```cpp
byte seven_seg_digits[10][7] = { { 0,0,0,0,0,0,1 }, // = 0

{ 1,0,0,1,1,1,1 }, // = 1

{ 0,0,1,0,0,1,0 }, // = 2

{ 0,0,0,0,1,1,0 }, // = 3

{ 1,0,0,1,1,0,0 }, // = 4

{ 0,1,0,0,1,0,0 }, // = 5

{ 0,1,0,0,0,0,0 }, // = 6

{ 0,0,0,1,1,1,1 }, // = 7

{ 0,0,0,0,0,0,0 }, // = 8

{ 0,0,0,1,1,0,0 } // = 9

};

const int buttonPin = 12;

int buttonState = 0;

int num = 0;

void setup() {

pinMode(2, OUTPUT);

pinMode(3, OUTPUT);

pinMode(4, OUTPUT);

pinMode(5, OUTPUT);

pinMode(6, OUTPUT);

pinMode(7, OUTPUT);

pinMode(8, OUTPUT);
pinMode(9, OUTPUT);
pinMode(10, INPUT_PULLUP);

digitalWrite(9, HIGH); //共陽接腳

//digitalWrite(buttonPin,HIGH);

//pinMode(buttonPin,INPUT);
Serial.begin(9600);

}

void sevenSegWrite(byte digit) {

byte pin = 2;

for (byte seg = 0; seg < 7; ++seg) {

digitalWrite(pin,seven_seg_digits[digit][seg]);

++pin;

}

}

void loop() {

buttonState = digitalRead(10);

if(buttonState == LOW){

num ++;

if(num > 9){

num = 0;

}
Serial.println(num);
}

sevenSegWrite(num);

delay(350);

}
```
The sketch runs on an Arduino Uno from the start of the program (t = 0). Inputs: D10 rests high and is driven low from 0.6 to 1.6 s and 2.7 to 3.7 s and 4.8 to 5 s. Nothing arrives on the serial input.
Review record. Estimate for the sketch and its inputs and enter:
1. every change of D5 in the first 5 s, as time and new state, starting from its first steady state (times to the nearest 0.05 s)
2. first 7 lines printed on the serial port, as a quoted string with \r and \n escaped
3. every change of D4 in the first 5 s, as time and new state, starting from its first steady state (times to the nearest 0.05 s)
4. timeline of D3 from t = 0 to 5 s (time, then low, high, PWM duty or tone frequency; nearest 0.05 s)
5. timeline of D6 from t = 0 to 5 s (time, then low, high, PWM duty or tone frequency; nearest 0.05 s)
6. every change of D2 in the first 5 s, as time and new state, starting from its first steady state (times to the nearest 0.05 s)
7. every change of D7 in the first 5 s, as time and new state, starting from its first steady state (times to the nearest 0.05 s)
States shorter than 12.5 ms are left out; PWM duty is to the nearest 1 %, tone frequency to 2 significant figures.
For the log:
0 s low; 0.7 s high; 1.05 s low; 2.8 s high; 3.15 s low; 4.9 s high
"1\r\n2\r\n3\r\n4\r\n5\r\n6\r\n7\r\n"
0 s low; 1.05 s high; 1.4 s low
0 s low; 3.15 s high; 4.9 s low
0 s low; 0.7 s high; 1.05 s low; 1.4 s high; 3.5 s low; 4.9 s high
0 s low; 0.7 s high; 1.05 s low; 2.8 s high; 3.15 s low
0 s low; 0.7 s high; 2.8 s low; 4.9 s high
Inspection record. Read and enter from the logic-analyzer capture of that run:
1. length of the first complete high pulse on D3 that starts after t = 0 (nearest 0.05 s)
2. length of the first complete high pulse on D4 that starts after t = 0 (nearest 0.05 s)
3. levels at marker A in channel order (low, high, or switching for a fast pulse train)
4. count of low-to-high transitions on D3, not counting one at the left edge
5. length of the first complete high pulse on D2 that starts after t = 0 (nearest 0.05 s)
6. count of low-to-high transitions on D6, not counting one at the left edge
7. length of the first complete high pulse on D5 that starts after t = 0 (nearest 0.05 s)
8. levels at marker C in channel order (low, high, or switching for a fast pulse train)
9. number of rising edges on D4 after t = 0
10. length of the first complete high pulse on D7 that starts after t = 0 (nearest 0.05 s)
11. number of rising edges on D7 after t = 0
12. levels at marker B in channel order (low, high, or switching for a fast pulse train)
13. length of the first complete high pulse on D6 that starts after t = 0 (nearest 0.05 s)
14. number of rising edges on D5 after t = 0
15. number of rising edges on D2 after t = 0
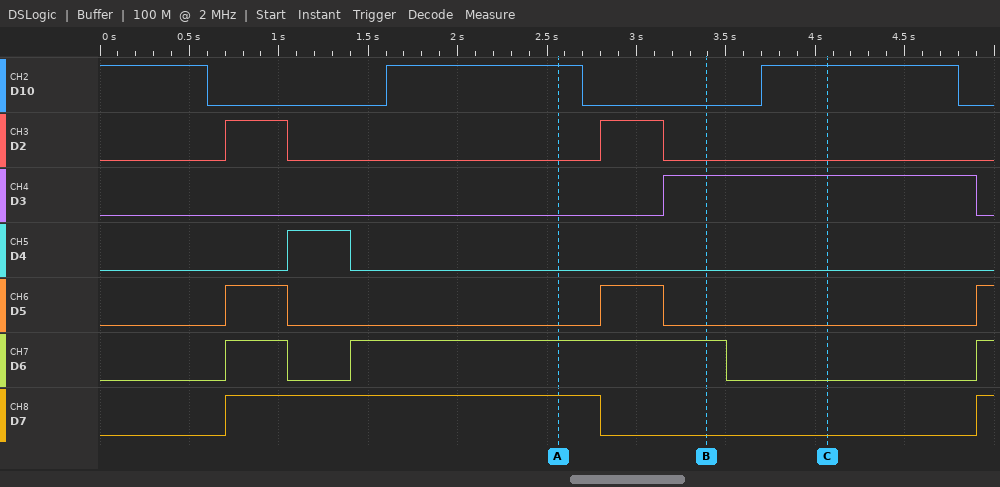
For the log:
1.75 s
0.35 s
D10 high, D2 low, D3 low, D4 low, D5 low, D6 high, D7 high
1
0.35 s
3
0.35 s
D10 high, D2 low, D3 high, D4 low, D5 low, D6 low, D7 low
1
2.10 s
2
D10 low, D2 low, D3 high, D4 low, D5 low, D6 high, D7 low
0.35 s
3
2
